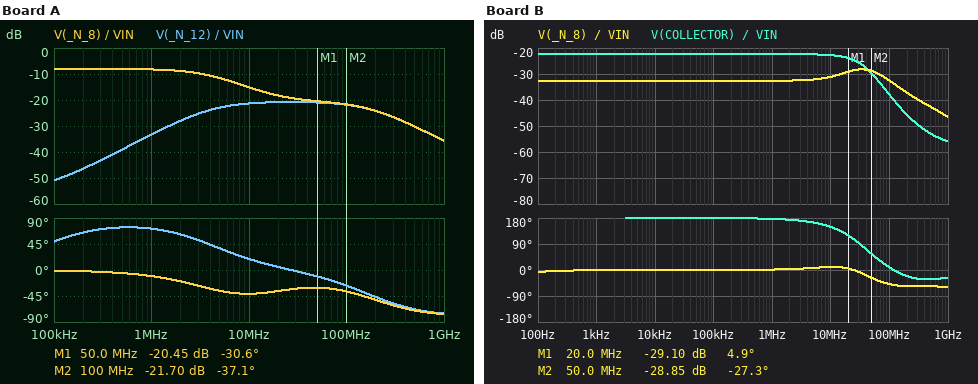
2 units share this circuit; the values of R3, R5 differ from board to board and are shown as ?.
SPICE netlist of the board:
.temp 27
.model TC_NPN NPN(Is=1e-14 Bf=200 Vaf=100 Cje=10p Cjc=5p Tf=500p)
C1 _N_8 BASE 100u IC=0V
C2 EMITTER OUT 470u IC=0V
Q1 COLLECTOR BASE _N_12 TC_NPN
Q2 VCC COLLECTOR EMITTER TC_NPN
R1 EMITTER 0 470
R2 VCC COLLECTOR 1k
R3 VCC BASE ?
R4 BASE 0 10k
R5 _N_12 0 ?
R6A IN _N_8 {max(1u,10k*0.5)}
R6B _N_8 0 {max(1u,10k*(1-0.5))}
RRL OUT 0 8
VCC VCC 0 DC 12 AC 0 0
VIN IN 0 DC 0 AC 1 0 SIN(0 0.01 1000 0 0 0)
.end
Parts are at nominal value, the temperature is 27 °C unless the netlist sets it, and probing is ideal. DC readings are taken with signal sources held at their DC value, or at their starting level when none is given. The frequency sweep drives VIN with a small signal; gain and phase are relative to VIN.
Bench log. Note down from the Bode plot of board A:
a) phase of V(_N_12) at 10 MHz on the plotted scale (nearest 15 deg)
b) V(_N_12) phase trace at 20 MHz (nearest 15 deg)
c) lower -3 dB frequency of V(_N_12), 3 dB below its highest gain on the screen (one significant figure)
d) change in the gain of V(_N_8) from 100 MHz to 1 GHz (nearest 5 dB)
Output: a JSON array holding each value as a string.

["15 deg", "0 deg", "4 MHz", "-15 dB"]
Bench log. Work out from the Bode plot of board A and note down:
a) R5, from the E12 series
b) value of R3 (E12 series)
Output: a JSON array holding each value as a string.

["680 Ω", "270 kΩ"]
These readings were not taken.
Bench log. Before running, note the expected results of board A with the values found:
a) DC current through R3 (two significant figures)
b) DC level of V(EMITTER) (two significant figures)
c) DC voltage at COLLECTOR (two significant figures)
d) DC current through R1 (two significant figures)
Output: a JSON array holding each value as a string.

["43 µA", "11 V", "12 V", "24 mA"]
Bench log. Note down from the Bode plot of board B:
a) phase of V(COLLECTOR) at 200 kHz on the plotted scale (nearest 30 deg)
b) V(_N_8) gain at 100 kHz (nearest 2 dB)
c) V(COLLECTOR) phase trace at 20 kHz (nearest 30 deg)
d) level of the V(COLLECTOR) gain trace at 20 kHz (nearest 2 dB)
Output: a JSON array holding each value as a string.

["180 deg", "-32 dB", "180 deg", "-22 dB"]
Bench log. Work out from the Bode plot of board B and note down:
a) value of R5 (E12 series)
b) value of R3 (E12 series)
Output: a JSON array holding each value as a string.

["82 Ω", "39 kΩ"]
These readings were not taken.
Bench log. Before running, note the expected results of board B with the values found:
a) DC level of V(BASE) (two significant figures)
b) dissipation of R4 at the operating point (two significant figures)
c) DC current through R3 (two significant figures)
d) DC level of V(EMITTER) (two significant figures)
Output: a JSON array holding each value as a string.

["1.6 V", "260 µW", "270 µA", "400 mV"]
